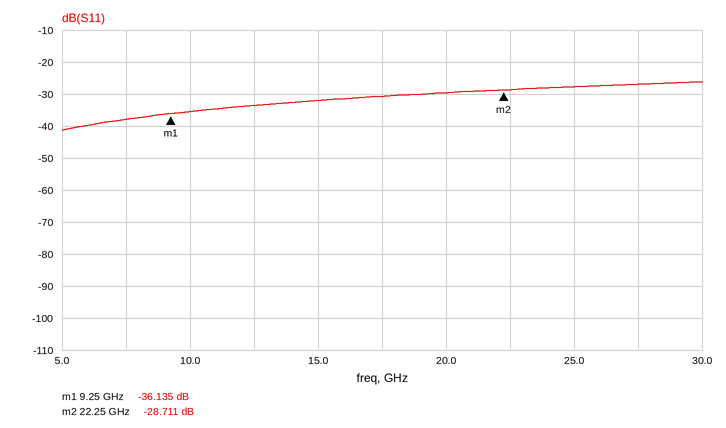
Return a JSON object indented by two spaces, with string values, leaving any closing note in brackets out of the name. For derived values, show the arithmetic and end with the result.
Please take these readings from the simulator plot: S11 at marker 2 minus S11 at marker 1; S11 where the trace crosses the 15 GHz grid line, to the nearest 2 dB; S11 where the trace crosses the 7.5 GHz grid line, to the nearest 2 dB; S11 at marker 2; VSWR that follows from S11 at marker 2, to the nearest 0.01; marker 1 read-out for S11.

{
  "S11 at marker 2 minus S11 at marker 1": "-28.711 − (-36.135) = 7.424 dB",
  "S11 where the trace crosses the 15 GHz grid line, to the nearest 2 dB": "-32 dB",
  "S11 where the trace crosses the 7.5 GHz grid line, to the nearest 2 dB": "-38 dB",
  "S11 at marker 2": "-28.711 dB",
  "VSWR that follows from S11 at marker 2, to the nearest 0.01": "(1 + 0.0367)/(1 − 0.0367) ≈ 1.08",
  "marker 1 read-out for S11": "-36.135 dB"
}
